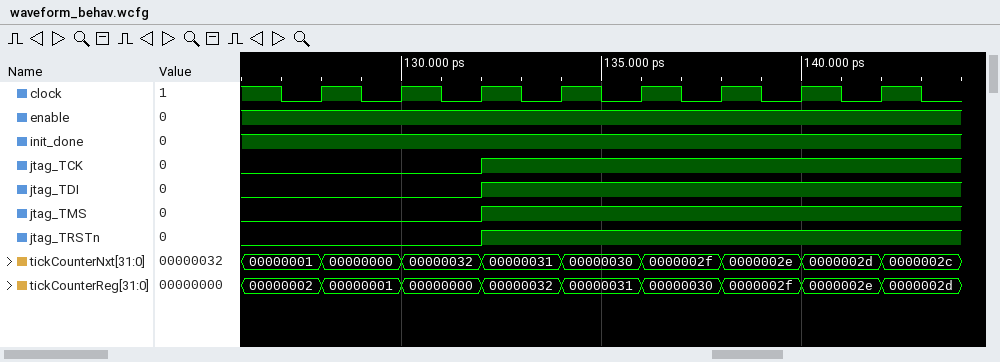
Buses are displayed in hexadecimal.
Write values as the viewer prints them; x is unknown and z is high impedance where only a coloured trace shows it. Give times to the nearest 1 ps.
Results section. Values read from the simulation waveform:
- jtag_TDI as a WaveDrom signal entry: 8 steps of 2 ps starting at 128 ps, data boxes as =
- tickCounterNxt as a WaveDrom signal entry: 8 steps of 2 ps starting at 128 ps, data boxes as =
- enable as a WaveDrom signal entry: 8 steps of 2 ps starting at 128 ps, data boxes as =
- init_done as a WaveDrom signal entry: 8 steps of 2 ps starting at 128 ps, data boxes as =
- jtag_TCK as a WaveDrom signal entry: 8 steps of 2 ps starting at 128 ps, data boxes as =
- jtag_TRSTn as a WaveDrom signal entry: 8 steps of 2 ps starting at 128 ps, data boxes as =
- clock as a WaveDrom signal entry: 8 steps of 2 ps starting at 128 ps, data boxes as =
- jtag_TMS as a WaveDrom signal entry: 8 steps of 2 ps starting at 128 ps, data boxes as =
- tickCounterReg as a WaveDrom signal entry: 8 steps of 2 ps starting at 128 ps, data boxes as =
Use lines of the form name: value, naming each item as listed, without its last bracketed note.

jtag_TDI as a WaveDrom signal entry: 8 steps of 2 ps starting at 128 ps, data boxes as =: {name: 'jtag_TDI', wave: '0.1.....'}
tickCounterNxt as a WaveDrom signal entry: 8 steps of 2 ps starting at 128 ps, data boxes as =: {name: 'tickCounterNxt', wave: '========', data: '00000000 00000032 00000031 00000030 0000002f 0000002e 0000002d 0000002c'}
enable as a WaveDrom signal entry: 8 steps of 2 ps starting at 128 ps, data boxes as =: {name: 'enable', wave: '1.......'}
init_done as a WaveDrom signal entry: 8 steps of 2 ps starting at 128 ps, data boxes as =: {name: 'init_done', wave: '1.......'}
jtag_TCK as a WaveDrom signal entry: 8 steps of 2 ps starting at 128 ps, data boxes as =: {name: 'jtag_TCK', wave: '0.1.....'}
jtag_TRSTn as a WaveDrom signal entry: 8 steps of 2 ps starting at 128 ps, data boxes as =: {name: 'jtag_TRSTn', wave: '0.1.....'}
clock as a WaveDrom signal entry: 8 steps of 2 ps starting at 128 ps, data boxes as =: {name: 'clock', wave: 'p.......'}
jtag_TMS as a WaveDrom signal entry: 8 steps of 2 ps starting at 128 ps, data boxes as =: {name: 'jtag_TMS', wave: '0.1.....'}
tickCounterReg as a WaveDrom signal entry: 8 steps of 2 ps starting at 128 ps, data boxes as =: {name: 'tickCounterReg', wave: '========', data: '00000001 00000000 00000032 00000031 00000030 0000002f 0000002e 0000002d'}
